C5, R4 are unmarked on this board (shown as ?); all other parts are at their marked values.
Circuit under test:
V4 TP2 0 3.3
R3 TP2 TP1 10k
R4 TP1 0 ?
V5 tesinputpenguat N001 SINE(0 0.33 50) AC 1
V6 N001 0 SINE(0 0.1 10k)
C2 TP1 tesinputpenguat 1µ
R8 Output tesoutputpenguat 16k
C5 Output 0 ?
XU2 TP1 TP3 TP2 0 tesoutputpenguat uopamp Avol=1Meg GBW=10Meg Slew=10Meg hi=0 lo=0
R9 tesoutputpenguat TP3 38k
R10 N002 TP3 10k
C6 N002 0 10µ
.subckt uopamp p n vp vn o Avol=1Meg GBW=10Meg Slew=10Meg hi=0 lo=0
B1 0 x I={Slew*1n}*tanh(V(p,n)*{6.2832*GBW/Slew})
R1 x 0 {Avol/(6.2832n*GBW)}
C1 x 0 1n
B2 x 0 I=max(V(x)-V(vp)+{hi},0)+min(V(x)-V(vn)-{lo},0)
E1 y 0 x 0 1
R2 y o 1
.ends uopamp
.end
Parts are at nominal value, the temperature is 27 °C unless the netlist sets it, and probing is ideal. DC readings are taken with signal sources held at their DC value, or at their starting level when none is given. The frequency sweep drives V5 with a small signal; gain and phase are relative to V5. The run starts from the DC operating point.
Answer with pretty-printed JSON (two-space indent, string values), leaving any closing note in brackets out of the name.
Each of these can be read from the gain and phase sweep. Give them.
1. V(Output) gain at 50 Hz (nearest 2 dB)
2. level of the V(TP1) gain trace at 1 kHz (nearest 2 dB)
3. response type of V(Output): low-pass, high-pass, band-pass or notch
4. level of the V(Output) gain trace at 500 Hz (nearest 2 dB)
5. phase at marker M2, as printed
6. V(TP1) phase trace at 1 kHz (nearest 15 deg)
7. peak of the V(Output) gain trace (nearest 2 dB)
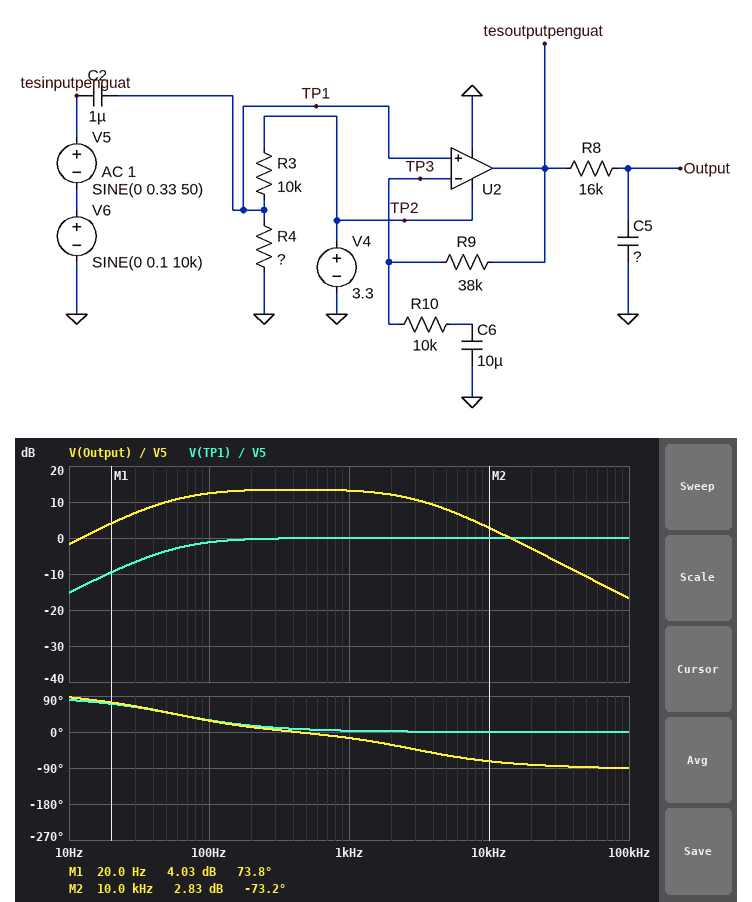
{
  "V(Output) gain at 50 Hz": "10 dB",
  "level of the V(TP1) gain trace at 1 kHz": "0 dB",
  "response type of V(Output): low-pass, high-pass, band-pass or notch": "band-pass",
  "level of the V(Output) gain trace at 500 Hz": "14 dB",
  "phase at marker M2, as printed": "-73.2 deg",
  "V(TP1) phase trace at 1 kHz": "0 deg",
  "peak of the V(Output) gain trace": "14 dB"
}
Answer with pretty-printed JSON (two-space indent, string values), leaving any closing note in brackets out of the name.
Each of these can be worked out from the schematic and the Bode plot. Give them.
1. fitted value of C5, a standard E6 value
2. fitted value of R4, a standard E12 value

{
  "fitted value of C5, a standard E6 value": "3.3 nF",
  "fitted value of R4, a standard E12 value": "3.9 kΩ"
}
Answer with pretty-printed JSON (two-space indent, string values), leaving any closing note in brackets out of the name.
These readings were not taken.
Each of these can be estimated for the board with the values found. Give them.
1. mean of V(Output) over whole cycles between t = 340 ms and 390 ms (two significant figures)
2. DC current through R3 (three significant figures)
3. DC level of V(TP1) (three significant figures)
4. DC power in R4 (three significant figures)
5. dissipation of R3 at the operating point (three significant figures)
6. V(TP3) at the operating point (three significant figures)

{
  "mean of V(Output) over whole cycles between t = 340 ms and 390 ms": "940 mV",
  "DC current through R3": "237 µA",
  "DC level of V(TP1)": "926 mV",
  "DC power in R4": "220 µW",
  "dissipation of R3 at the operating point": "564 µW",
  "V(TP3) at the operating point": "926 mV"
}
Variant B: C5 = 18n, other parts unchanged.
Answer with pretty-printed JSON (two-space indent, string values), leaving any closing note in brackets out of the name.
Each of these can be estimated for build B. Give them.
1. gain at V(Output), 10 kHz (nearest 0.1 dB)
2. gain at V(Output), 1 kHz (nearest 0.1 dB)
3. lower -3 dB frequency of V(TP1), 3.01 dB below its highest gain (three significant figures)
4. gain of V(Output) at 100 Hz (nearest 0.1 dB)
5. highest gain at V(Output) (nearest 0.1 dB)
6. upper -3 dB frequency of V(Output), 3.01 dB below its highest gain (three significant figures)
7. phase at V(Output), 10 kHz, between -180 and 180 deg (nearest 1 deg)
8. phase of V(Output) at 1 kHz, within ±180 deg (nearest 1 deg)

{
  "gain at V(Output), 10 kHz": "-11.5 dB",
  "gain at V(Output), 1 kHz": "7.3 dB",
  "lower -3 dB frequency of V(TP1), 3.01 dB below its highest gain": "56.7 Hz",
  "gain of V(Output) at 100 Hz": "12.3 dB",
  "highest gain at V(Output)": "12.8 dB",
  "upper -3 dB frequency of V(Output), 3.01 dB below its highest gain": "657 Hz",
  "phase at V(Output), 10 kHz, between -180 and 180 deg": "-87 deg",
  "phase of V(Output) at 1 kHz, within ±180 deg": "-58 deg"
}
